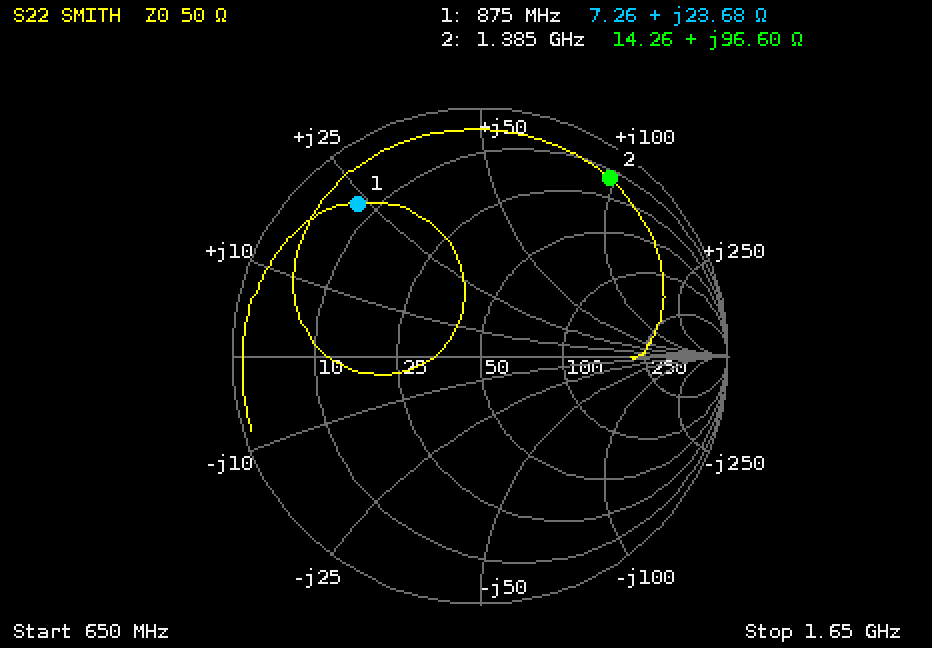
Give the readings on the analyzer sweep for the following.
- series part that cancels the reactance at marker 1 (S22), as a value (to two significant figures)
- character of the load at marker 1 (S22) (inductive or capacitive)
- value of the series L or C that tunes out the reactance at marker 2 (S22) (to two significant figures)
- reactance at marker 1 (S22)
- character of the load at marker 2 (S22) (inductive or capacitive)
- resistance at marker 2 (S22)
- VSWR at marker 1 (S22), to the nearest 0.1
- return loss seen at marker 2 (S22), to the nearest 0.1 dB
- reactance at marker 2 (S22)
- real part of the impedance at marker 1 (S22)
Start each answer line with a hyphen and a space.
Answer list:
- 7.7 pF
- inductive
- 1.2 pF
- +23.68 Ω
- inductive
- 14.26 Ω
- 8.5
- 1.0 dB
- +96.60 Ω
- 7.26 Ω
